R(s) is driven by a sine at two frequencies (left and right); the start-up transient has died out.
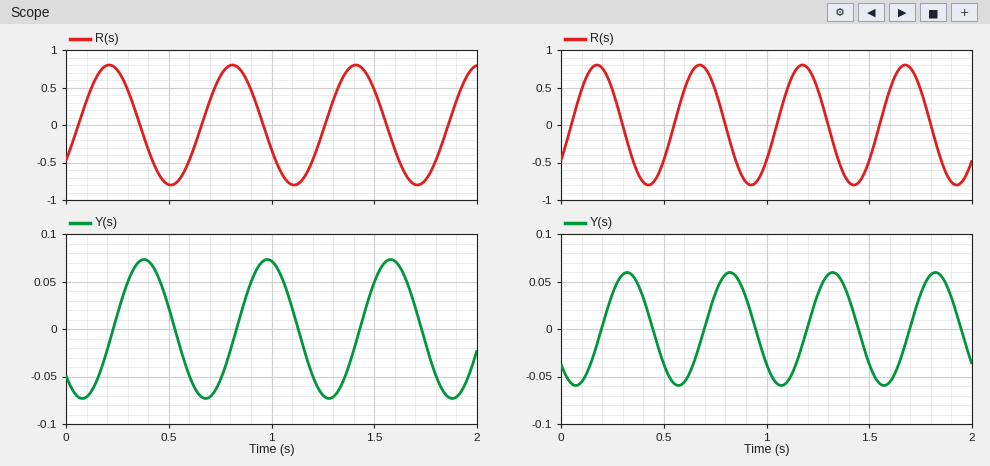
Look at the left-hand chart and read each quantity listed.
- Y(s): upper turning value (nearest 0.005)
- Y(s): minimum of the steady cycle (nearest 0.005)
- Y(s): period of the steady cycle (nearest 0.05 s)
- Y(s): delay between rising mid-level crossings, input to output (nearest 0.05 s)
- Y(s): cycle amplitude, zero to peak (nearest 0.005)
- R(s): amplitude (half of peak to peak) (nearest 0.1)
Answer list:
0.075
-0.075
0.60 s
0.15 s
0.075
0.8
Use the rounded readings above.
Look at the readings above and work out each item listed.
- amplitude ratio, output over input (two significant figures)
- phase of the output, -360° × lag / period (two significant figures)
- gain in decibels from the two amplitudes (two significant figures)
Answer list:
0.094
-90°
-21 dB
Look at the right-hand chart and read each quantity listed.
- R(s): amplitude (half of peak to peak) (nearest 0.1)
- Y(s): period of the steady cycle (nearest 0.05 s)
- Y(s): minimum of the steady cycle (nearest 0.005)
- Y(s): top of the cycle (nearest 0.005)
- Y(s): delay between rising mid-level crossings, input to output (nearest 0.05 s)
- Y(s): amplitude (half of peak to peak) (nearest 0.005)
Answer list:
0.8
0.50 s
-0.060
0.060
0.15 s
0.060
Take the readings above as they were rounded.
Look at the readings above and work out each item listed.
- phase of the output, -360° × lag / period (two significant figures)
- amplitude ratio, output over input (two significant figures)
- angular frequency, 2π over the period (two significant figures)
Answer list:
-110°
0.075
13 rad/s
